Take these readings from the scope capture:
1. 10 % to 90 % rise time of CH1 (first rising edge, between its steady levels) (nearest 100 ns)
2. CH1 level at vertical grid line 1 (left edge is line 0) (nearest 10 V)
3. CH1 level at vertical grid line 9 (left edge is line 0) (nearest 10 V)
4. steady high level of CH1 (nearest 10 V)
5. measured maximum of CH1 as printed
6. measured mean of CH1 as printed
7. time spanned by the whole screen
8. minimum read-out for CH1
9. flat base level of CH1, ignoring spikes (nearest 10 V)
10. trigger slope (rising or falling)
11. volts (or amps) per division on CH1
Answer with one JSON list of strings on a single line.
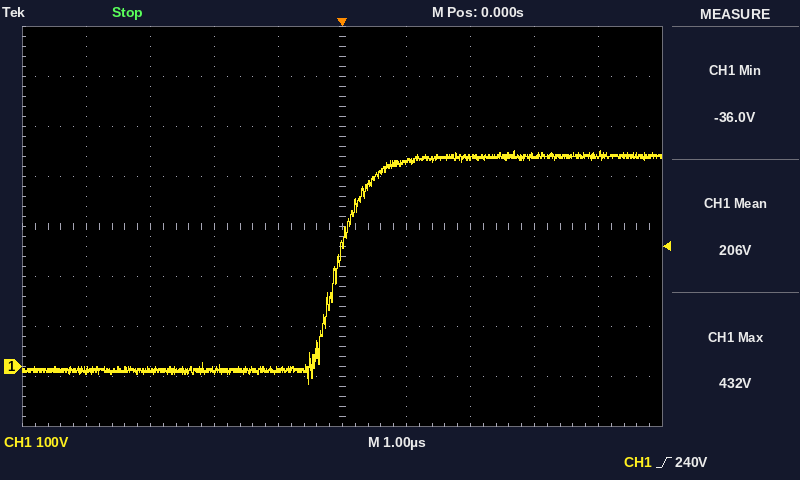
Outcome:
["900 ns", "-10 V", "420 V", "420 V", "432 V", "206 V", "10 µs", "-36.0 V", "-10 V", "rising", "100 V"]
